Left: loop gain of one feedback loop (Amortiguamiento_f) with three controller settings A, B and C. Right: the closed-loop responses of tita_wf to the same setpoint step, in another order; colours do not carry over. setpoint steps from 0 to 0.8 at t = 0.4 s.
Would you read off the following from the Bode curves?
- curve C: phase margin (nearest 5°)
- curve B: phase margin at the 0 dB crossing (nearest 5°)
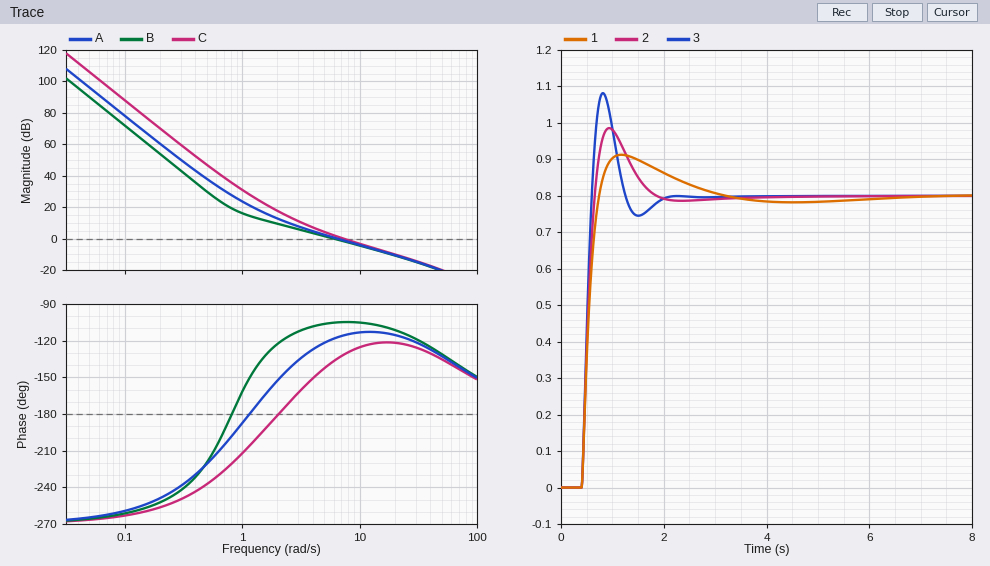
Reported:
50°
75°
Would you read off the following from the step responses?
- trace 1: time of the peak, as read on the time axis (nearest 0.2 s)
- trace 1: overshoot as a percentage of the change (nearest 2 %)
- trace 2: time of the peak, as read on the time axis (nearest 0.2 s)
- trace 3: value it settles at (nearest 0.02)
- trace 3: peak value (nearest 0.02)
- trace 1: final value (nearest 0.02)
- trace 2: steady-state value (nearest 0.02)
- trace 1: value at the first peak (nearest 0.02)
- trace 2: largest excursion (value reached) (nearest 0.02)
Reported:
1.2 s
14 %
1.0 s
0.80
1.08
0.80
0.80
0.92
0.98
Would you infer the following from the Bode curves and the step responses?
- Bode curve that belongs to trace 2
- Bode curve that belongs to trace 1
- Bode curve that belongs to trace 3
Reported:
A
B
C
